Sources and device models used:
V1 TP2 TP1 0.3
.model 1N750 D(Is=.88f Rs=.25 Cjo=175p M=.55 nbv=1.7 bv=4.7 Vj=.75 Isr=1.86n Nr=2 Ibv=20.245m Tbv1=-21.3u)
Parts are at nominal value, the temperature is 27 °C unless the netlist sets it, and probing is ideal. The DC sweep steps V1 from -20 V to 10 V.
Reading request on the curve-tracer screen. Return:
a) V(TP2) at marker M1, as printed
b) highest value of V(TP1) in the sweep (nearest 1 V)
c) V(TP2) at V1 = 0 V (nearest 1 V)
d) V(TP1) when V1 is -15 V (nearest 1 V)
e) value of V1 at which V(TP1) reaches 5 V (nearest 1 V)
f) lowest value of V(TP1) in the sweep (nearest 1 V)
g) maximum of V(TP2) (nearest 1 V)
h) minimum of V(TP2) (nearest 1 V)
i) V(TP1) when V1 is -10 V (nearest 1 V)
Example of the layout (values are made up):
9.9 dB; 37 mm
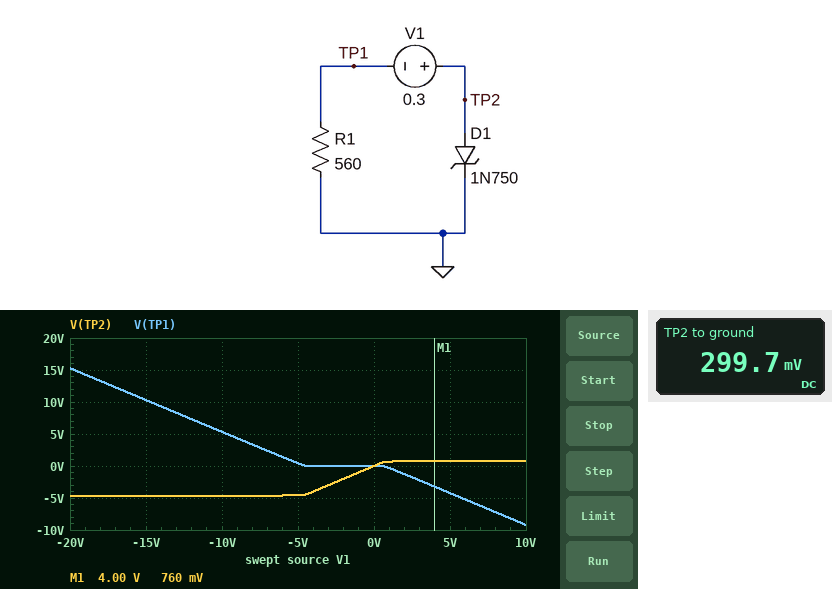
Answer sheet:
760 mV; 15 V; 0 V; 10 V; -10 V; -9 V; 1 V; -5 V; 5 V
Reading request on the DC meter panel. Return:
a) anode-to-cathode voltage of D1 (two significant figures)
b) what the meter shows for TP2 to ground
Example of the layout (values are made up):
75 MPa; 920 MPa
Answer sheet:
300 mV; 299.7 mV
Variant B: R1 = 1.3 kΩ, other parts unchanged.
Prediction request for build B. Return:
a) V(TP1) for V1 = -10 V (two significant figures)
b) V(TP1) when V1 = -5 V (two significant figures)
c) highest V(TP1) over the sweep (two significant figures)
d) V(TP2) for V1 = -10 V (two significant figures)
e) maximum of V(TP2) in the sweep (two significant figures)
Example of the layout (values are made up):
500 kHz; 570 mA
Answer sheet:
5.4 V; 480 mV; 15 V; -4.6 V; 770 mV
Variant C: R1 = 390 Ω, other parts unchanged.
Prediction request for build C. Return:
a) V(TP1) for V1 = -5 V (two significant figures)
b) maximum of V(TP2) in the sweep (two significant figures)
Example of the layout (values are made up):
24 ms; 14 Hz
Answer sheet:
430 mV; 800 mV
